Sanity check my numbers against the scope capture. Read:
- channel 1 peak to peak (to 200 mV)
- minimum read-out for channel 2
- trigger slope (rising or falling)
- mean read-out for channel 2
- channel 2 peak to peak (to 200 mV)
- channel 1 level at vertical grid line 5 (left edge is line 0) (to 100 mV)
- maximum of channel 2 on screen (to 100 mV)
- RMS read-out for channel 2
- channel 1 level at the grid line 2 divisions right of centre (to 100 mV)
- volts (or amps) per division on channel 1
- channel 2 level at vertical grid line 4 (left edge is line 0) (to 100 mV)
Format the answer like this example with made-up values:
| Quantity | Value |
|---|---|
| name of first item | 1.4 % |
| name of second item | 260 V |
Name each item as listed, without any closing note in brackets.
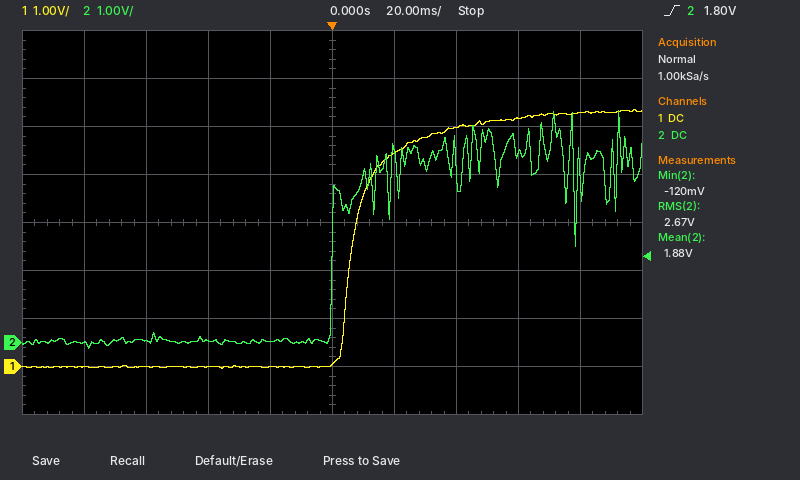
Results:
| Quantity | Value |
|---|---|
| channel 1 peak to peak | 5.4 V |
| minimum read-out for channel 2 | -120 mV |
| trigger slope | rising |
| mean read-out for channel 2 | 1.88 V |
| channel 2 peak to peak | 5.0 V |
| channel 1 level at vertical grid line 5 (left edge is line 0) | 100 mV |
| maximum of channel 2 on screen | 4.8 V |
| RMS read-out for channel 2 | 2.67 V |
| channel 1 level at the grid line 2 divisions right of centre | 5.0 V |
| volts (or amps) per division on channel 1 | 1 V |
| channel 2 level at vertical grid line 4 (left edge is line 0) | 0.0 V |
